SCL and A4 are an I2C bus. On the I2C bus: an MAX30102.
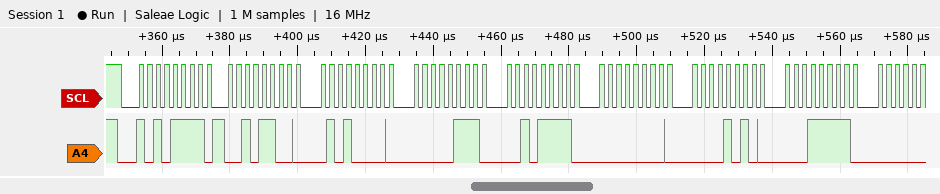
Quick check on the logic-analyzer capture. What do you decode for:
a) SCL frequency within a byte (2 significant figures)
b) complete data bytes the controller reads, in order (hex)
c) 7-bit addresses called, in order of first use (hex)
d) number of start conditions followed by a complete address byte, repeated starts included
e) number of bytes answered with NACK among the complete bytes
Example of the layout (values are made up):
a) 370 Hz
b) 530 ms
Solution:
a) 400 kHz
b) 2C 50 07 2F 00 0A 1F
c) 0x57
d) 1
e) 0
